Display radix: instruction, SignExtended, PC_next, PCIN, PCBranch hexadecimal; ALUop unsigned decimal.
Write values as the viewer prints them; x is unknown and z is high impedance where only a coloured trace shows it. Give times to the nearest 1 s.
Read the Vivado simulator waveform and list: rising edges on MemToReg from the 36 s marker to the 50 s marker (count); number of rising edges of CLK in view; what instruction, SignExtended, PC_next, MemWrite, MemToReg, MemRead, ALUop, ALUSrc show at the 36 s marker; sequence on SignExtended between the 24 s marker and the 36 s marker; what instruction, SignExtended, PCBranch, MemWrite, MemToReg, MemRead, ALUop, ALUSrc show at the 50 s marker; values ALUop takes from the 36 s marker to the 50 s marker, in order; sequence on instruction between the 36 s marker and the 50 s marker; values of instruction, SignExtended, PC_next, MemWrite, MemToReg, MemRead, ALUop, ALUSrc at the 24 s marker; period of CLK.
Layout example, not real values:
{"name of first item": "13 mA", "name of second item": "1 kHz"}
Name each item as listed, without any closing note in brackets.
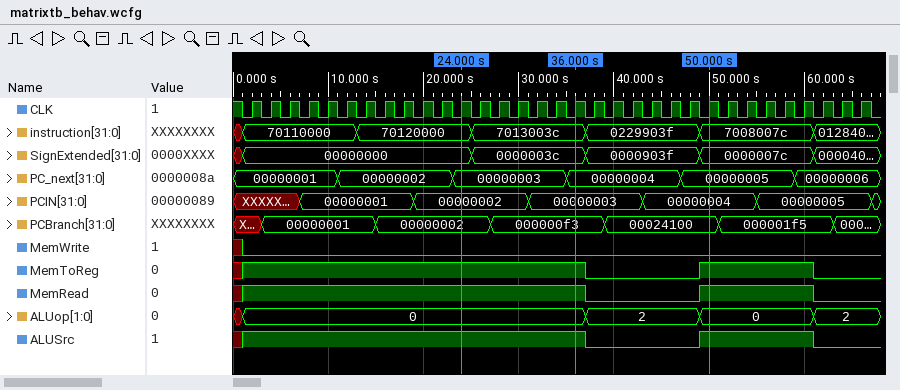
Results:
{"rising edges on MemToReg from the 36 s marker to the 50 s marker": "1", "number of rising edges of CLK in view": "33", "what instruction, SignExtended, PC_next, MemWrite, MemToReg, MemRead, ALUop, ALUSrc show at the 36 s marker": "instruction=7013003c, SignExtended=0000003c, PC_next=00000004, MemWrite=0, MemToReg=1, MemRead=1, ALUop=0, ALUSrc=1", "sequence on SignExtended between the 24 s marker and the 36 s marker": "00000000, 0000003c", "what instruction, SignExtended, PCBranch, MemWrite, MemToReg, MemRead, ALUop, ALUSrc show at the 50 s marker": "instruction=7008007c, SignExtended=0000007c, PCBranch=00024100, MemWrite=0, MemToReg=1, MemRead=1, ALUop=0, ALUSrc=1", "values ALUop takes from the 36 s marker to the 50 s marker, in order": "0, 2, 0", "sequence on instruction between the 36 s marker and the 50 s marker": "7013003c, 0229903f, 7008007c", "values of instruction, SignExtended, PC_next, MemWrite, MemToReg, MemRead, ALUop, ALUSrc at the 24 s marker": "instruction=70120000, SignExtended=00000000, PC_next=00000003, MemWrite=0, MemToReg=1, MemRead=1, ALUop=0, ALUSrc=1", "period of CLK": "2 s"}
